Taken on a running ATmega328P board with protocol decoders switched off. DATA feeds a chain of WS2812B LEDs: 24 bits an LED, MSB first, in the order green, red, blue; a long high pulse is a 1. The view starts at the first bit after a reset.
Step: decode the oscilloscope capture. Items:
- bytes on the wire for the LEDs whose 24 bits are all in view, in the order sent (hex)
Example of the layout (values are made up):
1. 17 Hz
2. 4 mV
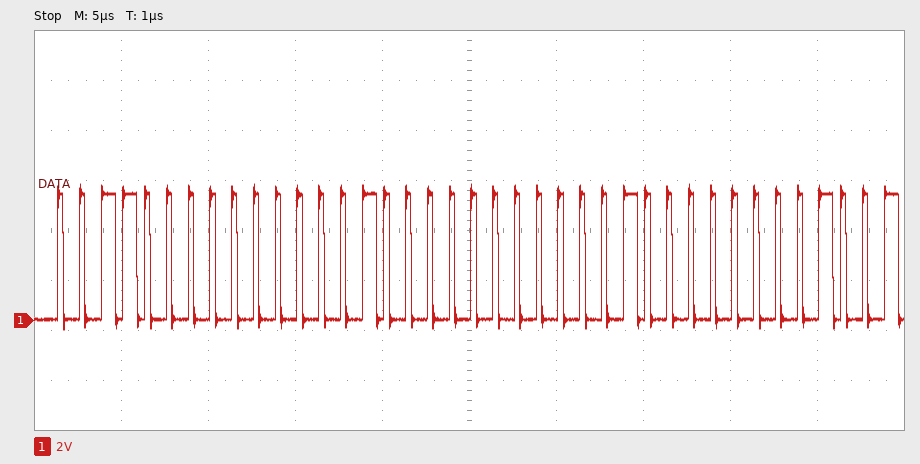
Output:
1. 30 02 00
